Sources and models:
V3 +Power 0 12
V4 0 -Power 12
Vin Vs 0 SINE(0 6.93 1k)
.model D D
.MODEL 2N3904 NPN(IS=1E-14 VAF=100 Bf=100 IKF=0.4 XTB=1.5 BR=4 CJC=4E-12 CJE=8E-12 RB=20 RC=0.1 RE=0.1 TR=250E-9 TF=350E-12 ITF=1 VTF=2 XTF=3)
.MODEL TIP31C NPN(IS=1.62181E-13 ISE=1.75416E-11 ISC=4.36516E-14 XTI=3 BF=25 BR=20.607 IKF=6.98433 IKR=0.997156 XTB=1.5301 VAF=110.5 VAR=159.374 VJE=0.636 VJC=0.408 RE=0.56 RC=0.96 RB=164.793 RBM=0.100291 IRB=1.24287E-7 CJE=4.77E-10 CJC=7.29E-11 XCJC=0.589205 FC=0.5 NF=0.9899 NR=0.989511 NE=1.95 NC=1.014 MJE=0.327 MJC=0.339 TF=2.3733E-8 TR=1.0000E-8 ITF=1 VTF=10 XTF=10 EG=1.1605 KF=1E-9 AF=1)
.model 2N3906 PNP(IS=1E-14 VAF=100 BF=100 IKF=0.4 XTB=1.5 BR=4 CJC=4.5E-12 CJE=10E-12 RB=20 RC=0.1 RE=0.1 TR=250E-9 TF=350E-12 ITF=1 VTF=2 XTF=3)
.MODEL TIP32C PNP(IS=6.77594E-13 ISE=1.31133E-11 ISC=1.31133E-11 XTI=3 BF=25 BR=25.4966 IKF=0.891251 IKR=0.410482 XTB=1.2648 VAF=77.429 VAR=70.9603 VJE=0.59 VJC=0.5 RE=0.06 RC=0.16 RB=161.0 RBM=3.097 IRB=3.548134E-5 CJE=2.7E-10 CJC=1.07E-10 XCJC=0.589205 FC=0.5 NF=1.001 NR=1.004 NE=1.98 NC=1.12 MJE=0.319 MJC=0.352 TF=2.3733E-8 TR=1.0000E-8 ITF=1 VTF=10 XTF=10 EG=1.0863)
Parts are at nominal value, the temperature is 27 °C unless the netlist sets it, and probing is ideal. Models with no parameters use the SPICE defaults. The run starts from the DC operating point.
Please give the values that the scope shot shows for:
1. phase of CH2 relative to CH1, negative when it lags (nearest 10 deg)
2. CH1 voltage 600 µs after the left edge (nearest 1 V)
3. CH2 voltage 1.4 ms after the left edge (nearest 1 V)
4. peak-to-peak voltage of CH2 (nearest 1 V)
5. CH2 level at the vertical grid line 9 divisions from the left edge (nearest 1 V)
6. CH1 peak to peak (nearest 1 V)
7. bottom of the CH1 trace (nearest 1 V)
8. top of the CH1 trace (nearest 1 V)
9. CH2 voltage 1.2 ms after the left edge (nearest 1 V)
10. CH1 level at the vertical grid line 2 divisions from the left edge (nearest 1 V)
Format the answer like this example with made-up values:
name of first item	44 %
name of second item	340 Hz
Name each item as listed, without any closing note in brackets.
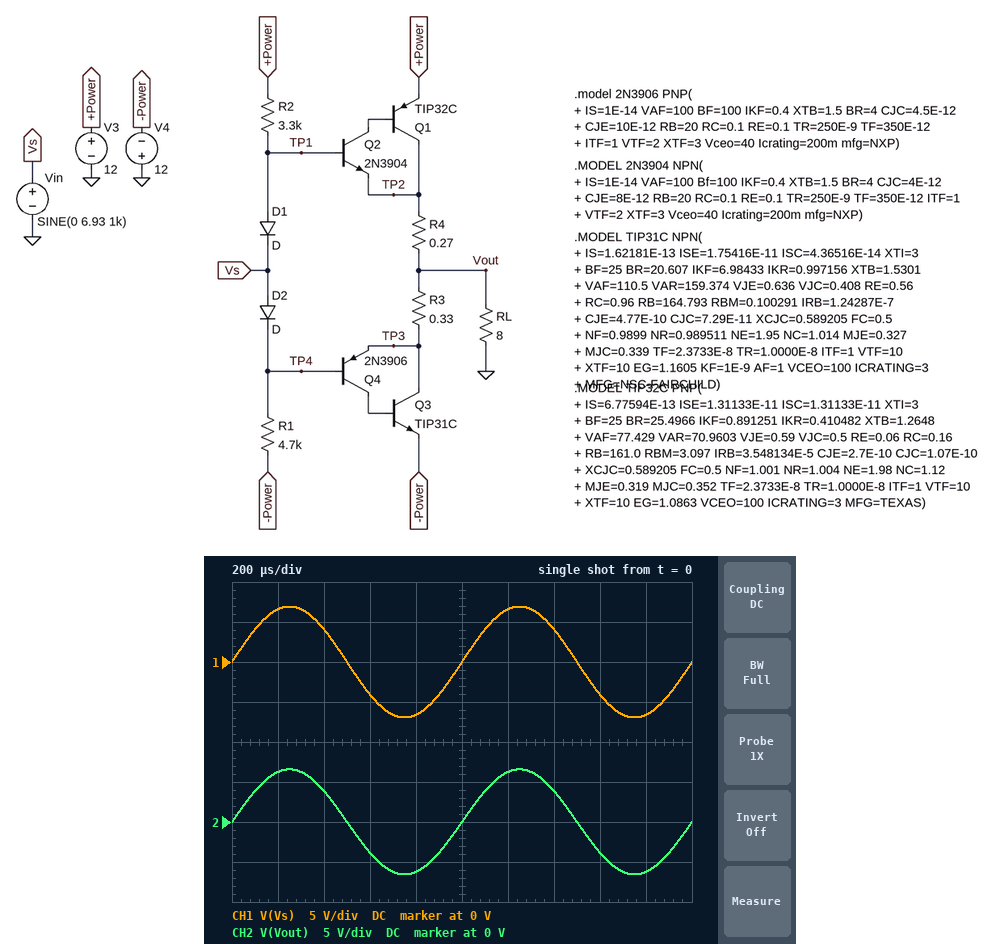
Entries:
phase of CH2 relative to CH1, negative when it lags	0 deg
CH1 voltage 600 µs after the left edge	-4 V
CH2 voltage 1.4 ms after the left edge	4 V
peak-to-peak voltage of CH2	13 V
CH2 level at the vertical grid line 9 divisions from the left edge	-6 V
CH1 peak to peak	14 V
bottom of the CH1 trace	-7 V
top of the CH1 trace	7 V
CH2 voltage 1.2 ms after the left edge	6 V
CH1 level at the vertical grid line 2 divisions from the left edge	4 V
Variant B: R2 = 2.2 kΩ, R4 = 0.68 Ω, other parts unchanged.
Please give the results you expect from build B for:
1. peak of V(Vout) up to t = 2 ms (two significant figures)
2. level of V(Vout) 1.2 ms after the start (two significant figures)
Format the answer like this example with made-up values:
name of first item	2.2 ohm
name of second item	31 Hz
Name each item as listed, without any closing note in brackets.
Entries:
peak of V(Vout) up to t = 2 ms	6.3 V
level of V(Vout) 1.2 ms after the start	6.0 V
